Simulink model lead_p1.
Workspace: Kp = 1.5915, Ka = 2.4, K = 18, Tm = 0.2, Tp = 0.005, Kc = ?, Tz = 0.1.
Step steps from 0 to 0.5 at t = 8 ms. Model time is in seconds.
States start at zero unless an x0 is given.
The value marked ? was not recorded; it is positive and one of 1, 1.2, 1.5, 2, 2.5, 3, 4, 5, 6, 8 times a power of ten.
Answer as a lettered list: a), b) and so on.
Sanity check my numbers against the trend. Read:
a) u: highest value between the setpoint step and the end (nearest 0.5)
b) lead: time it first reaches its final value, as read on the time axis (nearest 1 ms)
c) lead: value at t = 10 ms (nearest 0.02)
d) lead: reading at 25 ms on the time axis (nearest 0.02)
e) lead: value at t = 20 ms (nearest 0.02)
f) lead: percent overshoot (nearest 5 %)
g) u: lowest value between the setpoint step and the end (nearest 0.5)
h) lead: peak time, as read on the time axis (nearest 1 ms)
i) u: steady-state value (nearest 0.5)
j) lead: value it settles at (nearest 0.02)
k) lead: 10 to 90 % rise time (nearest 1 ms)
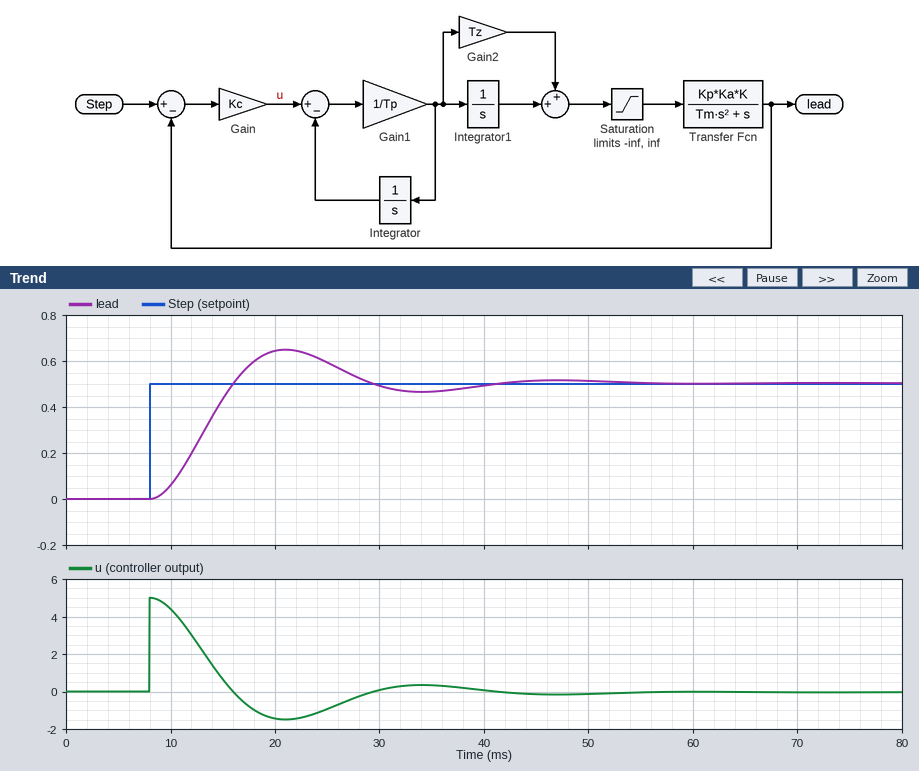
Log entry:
a) 5.0
b) 16 ms
c) 0.06
d) 0.60
e) 0.64
f) 30 %
g) -1.5
h) 21 ms
i) 0.0
j) 0.50
k) 5 ms
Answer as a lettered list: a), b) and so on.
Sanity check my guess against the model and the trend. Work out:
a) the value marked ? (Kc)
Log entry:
a) 10
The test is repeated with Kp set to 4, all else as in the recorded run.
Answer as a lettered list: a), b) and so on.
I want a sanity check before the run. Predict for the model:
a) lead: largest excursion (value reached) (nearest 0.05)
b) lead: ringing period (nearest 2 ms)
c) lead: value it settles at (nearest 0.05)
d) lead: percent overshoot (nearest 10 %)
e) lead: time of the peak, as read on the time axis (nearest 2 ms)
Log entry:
a) 0.75
b) 16 ms
c) 0.50
d) 50 %
e) 16 ms
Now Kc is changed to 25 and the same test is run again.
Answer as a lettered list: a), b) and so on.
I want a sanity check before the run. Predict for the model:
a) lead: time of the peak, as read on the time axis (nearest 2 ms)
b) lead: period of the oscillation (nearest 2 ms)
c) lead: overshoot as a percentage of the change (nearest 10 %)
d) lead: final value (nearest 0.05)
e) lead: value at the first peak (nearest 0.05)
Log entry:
a) 16 ms
b) 16 ms
c) 50 %
d) 0.50
e) 0.75
